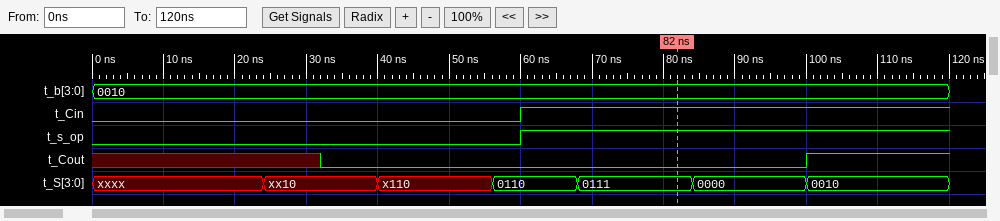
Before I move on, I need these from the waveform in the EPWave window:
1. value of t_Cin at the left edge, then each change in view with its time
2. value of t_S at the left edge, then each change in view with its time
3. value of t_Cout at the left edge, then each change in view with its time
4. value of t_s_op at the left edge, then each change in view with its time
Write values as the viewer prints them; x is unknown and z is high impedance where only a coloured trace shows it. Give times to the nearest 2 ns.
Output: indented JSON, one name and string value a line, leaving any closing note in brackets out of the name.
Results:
{
  "value of t_Cin at the left edge, then each change in view with its time": "0, 1 at 60 ns",
  "value of t_S at the left edge, then each change in view with its time": "xxxx, xx10 at 24 ns, x110 at 40 ns, 0110 at 56 ns, 0111 at 68 ns, 0000 at 84 ns, 0010 at 100 ns",
  "value of t_Cout at the left edge, then each change in view with its time": "x, 0 at 32 ns, 1 at 100 ns",
  "value of t_s_op at the left edge, then each change in view with its time": "0, 1 at 60 ns"
}
